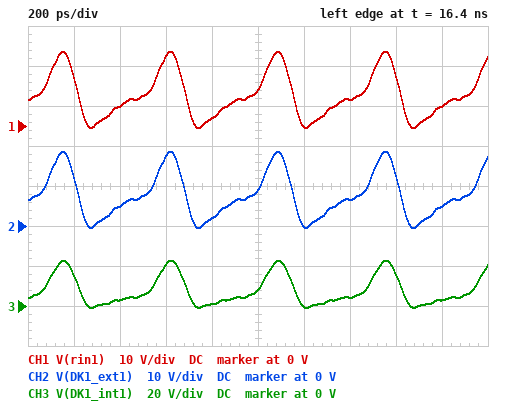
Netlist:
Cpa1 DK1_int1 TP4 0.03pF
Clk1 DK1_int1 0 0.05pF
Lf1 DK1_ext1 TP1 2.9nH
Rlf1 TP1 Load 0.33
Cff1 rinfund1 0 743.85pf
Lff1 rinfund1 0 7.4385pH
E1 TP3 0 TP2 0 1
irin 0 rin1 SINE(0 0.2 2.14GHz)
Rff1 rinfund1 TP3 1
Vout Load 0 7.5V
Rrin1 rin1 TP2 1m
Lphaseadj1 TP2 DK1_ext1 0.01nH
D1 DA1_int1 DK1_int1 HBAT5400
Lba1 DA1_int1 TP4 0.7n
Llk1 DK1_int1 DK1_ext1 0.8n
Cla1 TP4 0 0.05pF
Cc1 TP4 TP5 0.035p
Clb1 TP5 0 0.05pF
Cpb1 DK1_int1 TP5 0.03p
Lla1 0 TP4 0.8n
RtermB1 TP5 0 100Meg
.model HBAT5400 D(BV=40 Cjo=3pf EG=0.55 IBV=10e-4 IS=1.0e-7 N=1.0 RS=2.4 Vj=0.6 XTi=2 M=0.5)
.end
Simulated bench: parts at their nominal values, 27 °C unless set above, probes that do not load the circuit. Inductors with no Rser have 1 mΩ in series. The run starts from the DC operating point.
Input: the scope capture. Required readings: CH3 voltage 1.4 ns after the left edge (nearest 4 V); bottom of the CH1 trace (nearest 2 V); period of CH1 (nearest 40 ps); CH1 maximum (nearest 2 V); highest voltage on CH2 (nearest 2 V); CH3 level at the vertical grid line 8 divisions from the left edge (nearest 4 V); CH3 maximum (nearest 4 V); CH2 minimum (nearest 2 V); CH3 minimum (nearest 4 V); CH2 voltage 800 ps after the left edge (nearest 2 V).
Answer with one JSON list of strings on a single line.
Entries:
["4 V", "0 V", "480 ps", "18 V", "18 V", "16 V", "24 V", "0 V", "0 V", "2 V"]
